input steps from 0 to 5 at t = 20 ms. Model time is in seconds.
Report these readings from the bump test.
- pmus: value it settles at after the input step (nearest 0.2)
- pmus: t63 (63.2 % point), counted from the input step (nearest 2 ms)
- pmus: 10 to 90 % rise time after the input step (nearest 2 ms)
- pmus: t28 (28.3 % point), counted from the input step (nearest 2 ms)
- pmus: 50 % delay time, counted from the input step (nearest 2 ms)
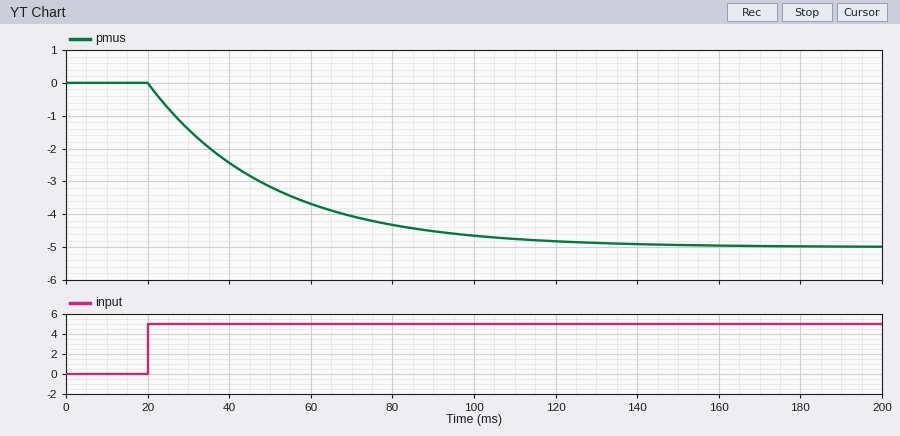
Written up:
-5.0
30 ms
66 ms
10 ms
20 ms
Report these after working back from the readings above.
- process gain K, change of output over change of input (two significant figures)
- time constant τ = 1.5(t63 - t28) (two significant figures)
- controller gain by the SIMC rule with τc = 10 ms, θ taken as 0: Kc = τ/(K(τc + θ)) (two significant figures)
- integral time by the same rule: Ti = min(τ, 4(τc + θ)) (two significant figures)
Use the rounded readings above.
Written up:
-1.0
30 ms
-3.0
30 ms
